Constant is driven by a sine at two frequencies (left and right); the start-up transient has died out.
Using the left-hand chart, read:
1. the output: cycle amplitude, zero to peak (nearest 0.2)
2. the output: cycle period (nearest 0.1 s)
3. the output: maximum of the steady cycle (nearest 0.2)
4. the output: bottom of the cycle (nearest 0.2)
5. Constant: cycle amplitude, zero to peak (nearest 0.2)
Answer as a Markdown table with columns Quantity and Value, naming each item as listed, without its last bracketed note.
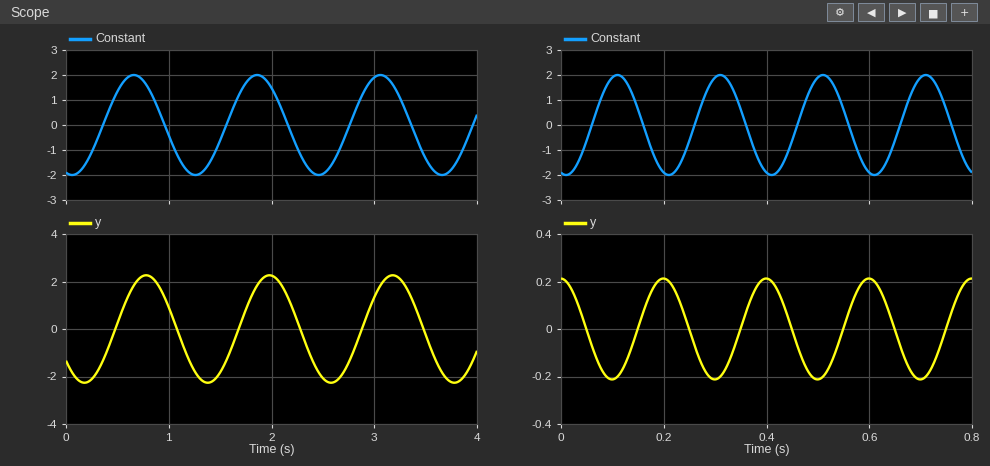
| Quantity | Value |
|---|---|
| the output: cycle amplitude, zero to peak | 2.2 |
| the output: cycle period | 1.2 s |
| the output: maximum of the steady cycle | 2.2 |
| the output: bottom of the cycle | -2.2 |
| Constant: cycle amplitude, zero to peak | 2.0 |
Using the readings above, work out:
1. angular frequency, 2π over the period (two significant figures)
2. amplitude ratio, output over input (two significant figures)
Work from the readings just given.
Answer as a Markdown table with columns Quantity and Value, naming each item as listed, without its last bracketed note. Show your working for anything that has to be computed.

| Quantity | Value |
|---|---|
| angular frequency, 2π over the period | 2π / 1.2 = 5.2 rad/s |
| amplitude ratio, output over input | 2.2 / 2 = 1.1 |
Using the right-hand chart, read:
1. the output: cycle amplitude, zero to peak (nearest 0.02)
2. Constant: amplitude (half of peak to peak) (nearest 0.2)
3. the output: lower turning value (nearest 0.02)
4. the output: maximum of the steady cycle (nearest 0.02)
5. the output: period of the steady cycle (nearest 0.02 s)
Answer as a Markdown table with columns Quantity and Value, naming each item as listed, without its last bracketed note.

| Quantity | Value |
|---|---|
| the output: cycle amplitude, zero to peak | 0.22 |
| Constant: amplitude (half of peak to peak) | 2.0 |
| the output: lower turning value | -0.22 |
| the output: maximum of the steady cycle | 0.22 |
| the output: period of the steady cycle | 0.20 s |
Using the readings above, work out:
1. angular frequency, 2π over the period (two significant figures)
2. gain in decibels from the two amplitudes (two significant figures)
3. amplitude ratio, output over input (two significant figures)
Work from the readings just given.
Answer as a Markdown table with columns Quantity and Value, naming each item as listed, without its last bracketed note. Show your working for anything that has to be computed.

| Quantity | Value |
|---|---|
| angular frequency, 2π over the period | 2π / 0.2 = 31 rad/s |
| gain in decibels from the two amplitudes | 20 log10(0.22 / 2) = -19 dB |
| amplitude ratio, output over input | 0.22 / 2 = 0.11 |
